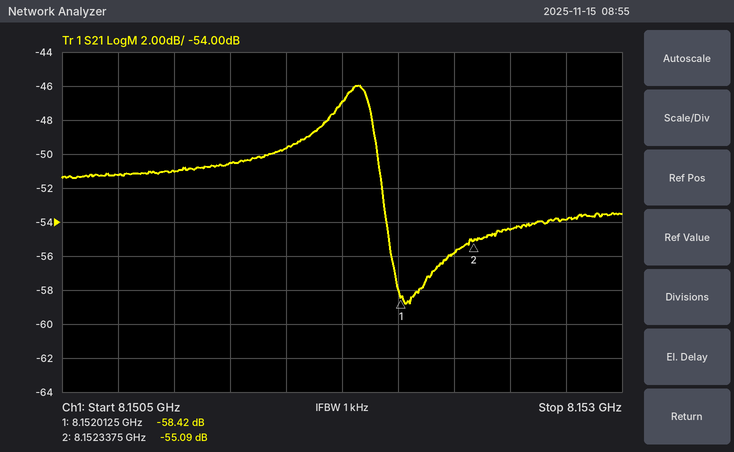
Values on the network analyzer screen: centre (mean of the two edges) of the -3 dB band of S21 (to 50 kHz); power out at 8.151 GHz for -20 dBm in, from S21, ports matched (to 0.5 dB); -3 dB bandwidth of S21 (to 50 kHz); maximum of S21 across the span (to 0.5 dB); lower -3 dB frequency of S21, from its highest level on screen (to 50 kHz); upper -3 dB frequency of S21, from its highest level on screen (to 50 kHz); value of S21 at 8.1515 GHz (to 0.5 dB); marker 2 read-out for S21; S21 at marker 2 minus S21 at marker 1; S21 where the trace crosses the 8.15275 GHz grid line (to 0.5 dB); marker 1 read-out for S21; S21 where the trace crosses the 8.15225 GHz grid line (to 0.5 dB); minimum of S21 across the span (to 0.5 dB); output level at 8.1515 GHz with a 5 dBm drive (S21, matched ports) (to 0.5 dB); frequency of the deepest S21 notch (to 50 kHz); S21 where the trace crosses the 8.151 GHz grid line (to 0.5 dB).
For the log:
8.15175 GHz
-71.0 dBm
300 kHz
-46.0 dB
8.15160 GHz
8.15190 GHz
-49.5 dB
-55.09 dB
3.33 dB
-54.0 dB
-58.42 dB
-56.0 dB
-59.0 dB
-44.5 dBm
8.15205 GHz
-51.0 dB
